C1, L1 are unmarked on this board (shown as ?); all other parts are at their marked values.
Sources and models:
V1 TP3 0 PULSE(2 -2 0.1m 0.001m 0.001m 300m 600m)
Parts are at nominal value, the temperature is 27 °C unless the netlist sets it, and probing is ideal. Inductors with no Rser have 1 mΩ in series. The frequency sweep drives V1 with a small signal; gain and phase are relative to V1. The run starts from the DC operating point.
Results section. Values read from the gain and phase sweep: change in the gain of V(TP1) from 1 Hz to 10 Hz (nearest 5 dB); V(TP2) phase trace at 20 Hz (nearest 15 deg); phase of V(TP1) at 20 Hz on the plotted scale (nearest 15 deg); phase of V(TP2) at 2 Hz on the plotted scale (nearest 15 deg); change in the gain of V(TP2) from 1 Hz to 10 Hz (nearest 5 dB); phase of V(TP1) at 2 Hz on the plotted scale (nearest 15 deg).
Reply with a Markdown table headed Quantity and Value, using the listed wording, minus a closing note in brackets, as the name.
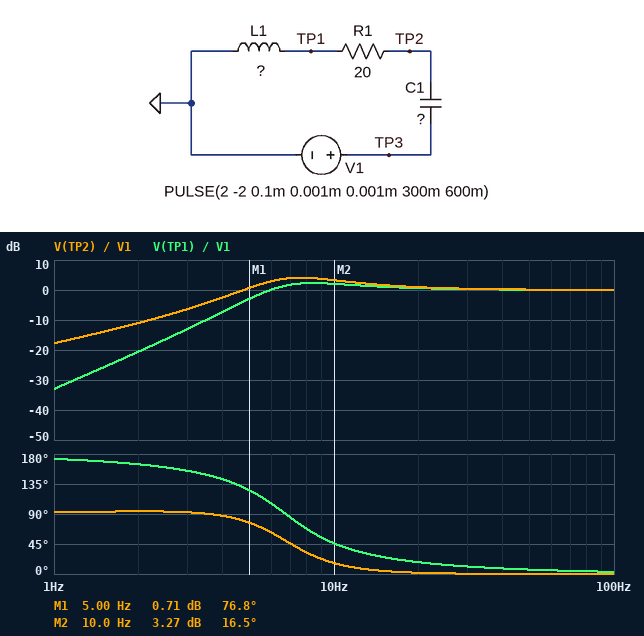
| Quantity | Value |
|---|---|
| change in the gain of V(TP1) from 1 Hz to 10 Hz | 35 dB |
| V(TP2) phase trace at 20 Hz | 0 deg |
| phase of V(TP1) at 20 Hz on the plotted scale | 15 deg |
| phase of V(TP2) at 2 Hz on the plotted scale | 90 deg |
| change in the gain of V(TP2) from 1 Hz to 10 Hz | 20 dB |
| phase of V(TP1) at 2 Hz on the plotted scale | 165 deg |
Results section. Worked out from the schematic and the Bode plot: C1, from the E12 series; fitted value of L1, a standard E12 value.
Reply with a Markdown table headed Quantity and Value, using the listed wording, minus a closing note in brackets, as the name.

| Quantity | Value |
|---|---|
| C1, from the E12 series | 1 mF |
| fitted value of L1, a standard E12 value | 560 mH |
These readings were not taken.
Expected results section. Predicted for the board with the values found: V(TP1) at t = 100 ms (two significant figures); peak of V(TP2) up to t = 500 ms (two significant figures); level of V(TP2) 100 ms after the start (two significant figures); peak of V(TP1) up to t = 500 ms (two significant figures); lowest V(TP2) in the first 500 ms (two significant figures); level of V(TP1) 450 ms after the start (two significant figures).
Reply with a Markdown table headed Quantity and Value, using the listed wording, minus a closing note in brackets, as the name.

| Quantity | Value |
|---|---|
| V(TP1) at t = 100 ms | 320 mV |
| peak of V(TP2) up to t = 500 ms | 4.0 V |
| level of V(TP2) 100 ms after the start | 720 mV |
| peak of V(TP1) up to t = 500 ms | 4.0 V |
| lowest V(TP2) in the first 500 ms | -4.0 V |
| level of V(TP1) 450 ms after the start | 300 mV |
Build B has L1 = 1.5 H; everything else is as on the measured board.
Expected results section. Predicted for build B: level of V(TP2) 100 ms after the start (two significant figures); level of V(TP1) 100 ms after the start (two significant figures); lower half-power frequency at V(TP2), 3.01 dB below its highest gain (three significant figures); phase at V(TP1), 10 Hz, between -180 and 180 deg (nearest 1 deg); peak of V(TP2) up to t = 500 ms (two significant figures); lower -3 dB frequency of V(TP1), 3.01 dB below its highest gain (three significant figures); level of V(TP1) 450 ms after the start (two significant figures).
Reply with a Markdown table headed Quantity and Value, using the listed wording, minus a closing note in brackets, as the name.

| Quantity | Value |
|---|---|
| level of V(TP2) 100 ms after the start | 1.3 V |
| level of V(TP1) 100 ms after the start | 2.0 V |
| lower half-power frequency at V(TP2), 3.01 dB below its highest gain | 3.45 Hz |
| phase at V(TP1), 10 Hz, between -180 and 180 deg | 14 deg |
| peak of V(TP2) up to t = 500 ms | 3.7 V |
| lower -3 dB frequency of V(TP1), 3.01 dB below its highest gain | 3.52 Hz |
| level of V(TP1) 450 ms after the start | -1.1 V |
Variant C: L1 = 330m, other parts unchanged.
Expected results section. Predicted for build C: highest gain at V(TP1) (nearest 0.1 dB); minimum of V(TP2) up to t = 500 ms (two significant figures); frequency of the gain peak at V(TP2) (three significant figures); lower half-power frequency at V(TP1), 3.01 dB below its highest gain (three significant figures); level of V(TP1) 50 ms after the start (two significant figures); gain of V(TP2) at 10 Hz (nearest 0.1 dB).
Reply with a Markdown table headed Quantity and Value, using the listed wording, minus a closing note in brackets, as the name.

| Quantity | Value |
|---|---|
| highest gain at V(TP1) | 0.7 dB |
| minimum of V(TP2) up to t = 500 ms | -4.0 V |
| frequency of the gain peak at V(TP2) | 10.5 Hz |
| lower half-power frequency at V(TP1), 3.01 dB below its highest gain | 7.65 Hz |
| level of V(TP1) 50 ms after the start | 1.0 V |
| gain of V(TP2) at 10 Hz | 2.9 dB |
